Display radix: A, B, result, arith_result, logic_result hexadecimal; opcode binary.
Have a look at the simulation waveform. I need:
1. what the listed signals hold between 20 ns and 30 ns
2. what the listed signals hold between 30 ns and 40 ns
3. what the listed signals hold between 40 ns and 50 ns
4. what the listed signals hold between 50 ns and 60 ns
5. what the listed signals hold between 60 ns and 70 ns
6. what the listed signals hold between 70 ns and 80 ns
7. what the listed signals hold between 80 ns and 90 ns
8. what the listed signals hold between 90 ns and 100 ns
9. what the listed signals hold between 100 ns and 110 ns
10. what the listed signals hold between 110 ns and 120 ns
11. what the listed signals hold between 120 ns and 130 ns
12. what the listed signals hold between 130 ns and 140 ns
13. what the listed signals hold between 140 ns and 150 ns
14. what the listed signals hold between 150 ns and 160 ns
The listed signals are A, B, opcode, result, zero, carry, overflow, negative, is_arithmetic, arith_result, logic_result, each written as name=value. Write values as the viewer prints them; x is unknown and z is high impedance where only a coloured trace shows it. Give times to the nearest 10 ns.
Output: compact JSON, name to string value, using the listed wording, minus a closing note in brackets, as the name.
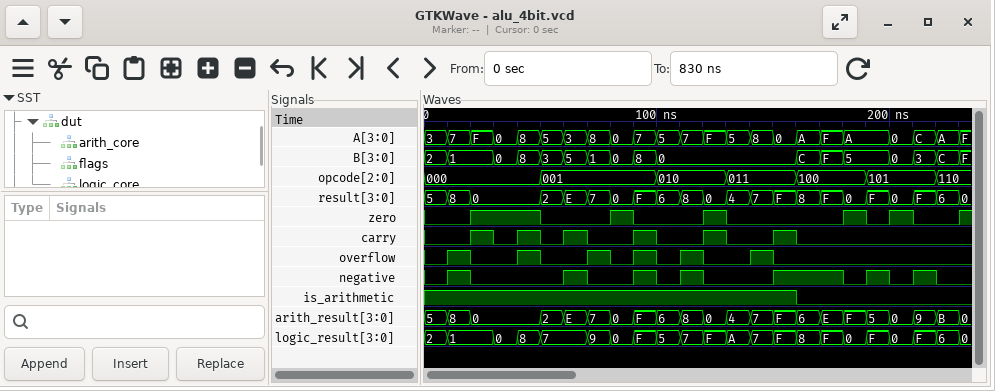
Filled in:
{"what the listed signals hold between 20 ns and 30 ns": "A=F, B=1, opcode=000, result=0, zero=1, carry=1, overflow=0, negative=0, is_arithmetic=1, arith_result=0, logic_result=1", "what the listed signals hold between 30 ns and 40 ns": "A=0, B=0, opcode=000, result=0, zero=1, carry=0, overflow=0, negative=0, is_arithmetic=1, arith_result=0, logic_result=0", "what the listed signals hold between 40 ns and 50 ns": "A=8, B=8, opcode=000, result=0, zero=1, carry=1, overflow=1, negative=0, is_arithmetic=1, arith_result=0, logic_result=8", "what the listed signals hold between 50 ns and 60 ns": "A=5, B=3, opcode=001, result=2, zero=0, carry=0, overflow=0, negative=0, is_arithmetic=1, arith_result=2, logic_result=7", "what the listed signals hold between 60 ns and 70 ns": "A=3, B=5, opcode=001, result=E, zero=0, carry=1, overflow=0, negative=1, is_arithmetic=1, arith_result=E, logic_result=7", "what the listed signals hold between 70 ns and 80 ns": "A=8, B=1, opcode=001, result=7, zero=0, carry=0, overflow=1, negative=0, is_arithmetic=1, arith_result=7, logic_result=9", "what the listed signals hold between 80 ns and 90 ns": "A=0, B=0, opcode=001, result=0, zero=1, carry=0, overflow=0, negative=0, is_arithmetic=1, arith_result=0, logic_result=0", "what the listed signals hold between 90 ns and 100 ns": "A=7, B=8, opcode=001, result=F, zero=0, carry=1, overflow=1, negative=1, is_arithmetic=1, arith_result=F, logic_result=F", "what the listed signals hold between 100 ns and 110 ns": "A=5, B=0, opcode=010, result=6, zero=0, carry=0, overflow=0, negative=0, is_arithmetic=1, arith_result=6, logic_result=5", "what the listed signals hold between 110 ns and 120 ns": "A=7, B=0, opcode=010, result=8, zero=0, carry=0, overflow=1, negative=1, is_arithmetic=1, arith_result=8, logic_result=7", "what the listed signals hold between 120 ns and 130 ns": "A=F, B=0, opcode=010, result=0, zero=1, carry=1, overflow=0, negative=0, is_arithmetic=1, arith_result=0, logic_result=F", "what the listed signals hold between 130 ns and 140 ns": "A=5, B=0, opcode=011, result=4, zero=0, carry=0, overflow=0, negative=0, is_arithmetic=1, arith_result=4, logic_result=A", "what the listed signals hold between 140 ns and 150 ns": "A=8, B=0, opcode=011, result=7, zero=0, carry=0, overflow=1, negative=0, is_arithmetic=1, arith_result=7, logic_result=7", "what the listed signals hold between 150 ns and 160 ns": "A=0, B=0, opcode=011, result=F, zero=0, carry=1, overflow=0, negative=1, is_arithmetic=1, arith_result=F, logic_result=F"}
